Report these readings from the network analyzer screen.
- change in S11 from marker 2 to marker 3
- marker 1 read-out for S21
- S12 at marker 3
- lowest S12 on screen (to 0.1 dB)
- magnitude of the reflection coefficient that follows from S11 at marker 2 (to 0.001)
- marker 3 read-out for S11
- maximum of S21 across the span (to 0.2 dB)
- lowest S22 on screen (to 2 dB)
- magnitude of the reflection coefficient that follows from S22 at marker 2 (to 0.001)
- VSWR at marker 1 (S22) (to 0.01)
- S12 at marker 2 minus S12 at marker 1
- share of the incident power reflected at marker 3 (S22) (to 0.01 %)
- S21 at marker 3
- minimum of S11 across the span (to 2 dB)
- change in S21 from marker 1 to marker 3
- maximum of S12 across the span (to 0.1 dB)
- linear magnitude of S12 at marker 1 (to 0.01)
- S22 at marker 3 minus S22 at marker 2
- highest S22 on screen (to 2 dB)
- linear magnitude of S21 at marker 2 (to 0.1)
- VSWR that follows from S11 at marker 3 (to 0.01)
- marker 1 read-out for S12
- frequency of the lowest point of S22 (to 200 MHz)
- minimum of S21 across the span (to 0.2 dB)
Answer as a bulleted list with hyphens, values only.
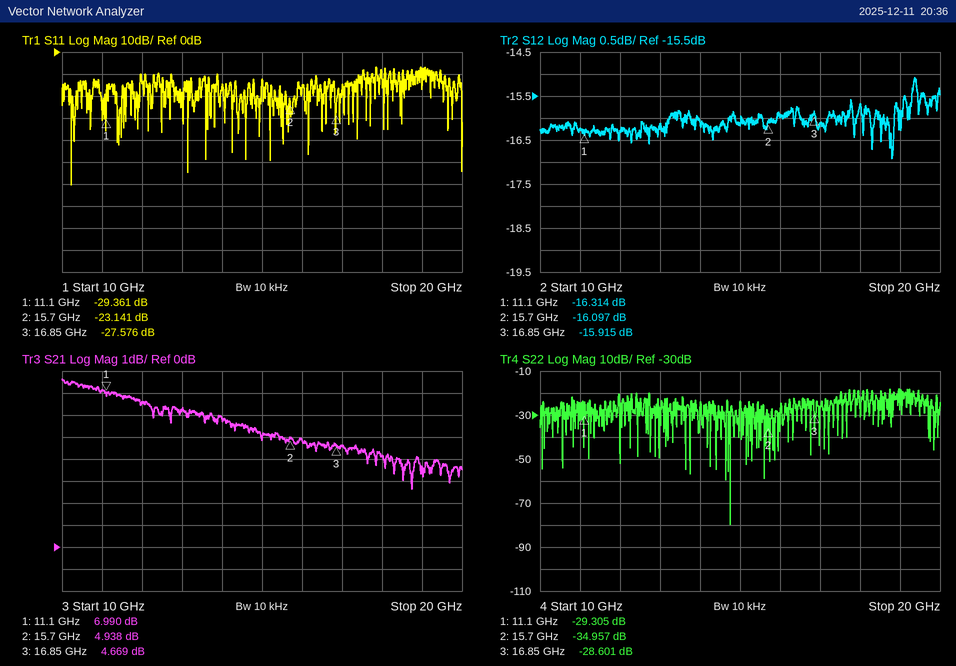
- -4.435 dB
- 6.990 dB
- -15.915 dB
- -16.9 dB
- 0.070
- -27.576 dB
- 7.6 dB
- -80 dB
- 0.018
- 1.07
- 0.217 dB
- 0.14 %
- 4.669 dB
- -60 dB
- -2.321 dB
- -15.1 dB
- 0.15
- 6.356 dB
- -18 dB
- 1.8
- 1.09
- -16.314 dB
- 14.8 GHz
- 2.6 dB
